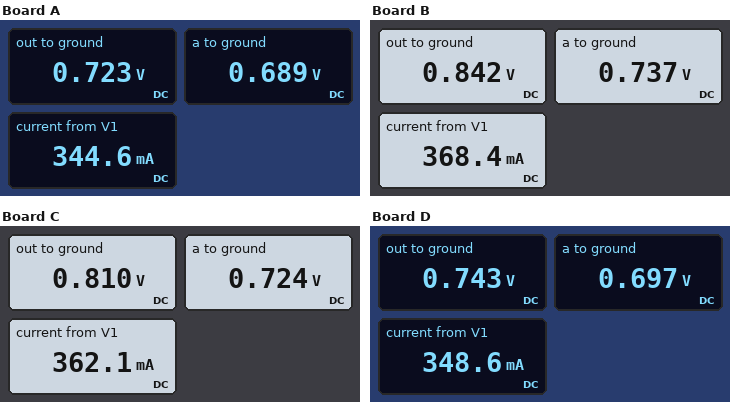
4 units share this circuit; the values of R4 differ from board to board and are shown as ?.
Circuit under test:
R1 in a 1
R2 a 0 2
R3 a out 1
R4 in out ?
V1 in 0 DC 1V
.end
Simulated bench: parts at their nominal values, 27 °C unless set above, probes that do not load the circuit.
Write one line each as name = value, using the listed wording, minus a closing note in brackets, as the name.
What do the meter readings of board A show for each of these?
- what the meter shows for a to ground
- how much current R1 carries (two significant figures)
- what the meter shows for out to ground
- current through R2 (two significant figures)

what the meter shows for a to ground = 0.689 V
how much current R1 carries = 310 mA
what the meter shows for out to ground = 0.723 V
current through R2 = 340 mA
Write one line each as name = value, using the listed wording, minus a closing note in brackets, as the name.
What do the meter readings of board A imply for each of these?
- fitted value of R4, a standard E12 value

fitted value of R4, a standard E12 value = 8.2 Ω
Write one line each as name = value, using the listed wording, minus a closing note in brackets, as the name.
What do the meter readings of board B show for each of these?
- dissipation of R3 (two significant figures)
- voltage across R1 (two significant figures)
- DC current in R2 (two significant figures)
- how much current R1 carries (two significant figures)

dissipation of R3 = 11 mW
voltage across R1 = 260 mV
DC current in R2 = 370 mA
how much current R1 carries = 260 mA
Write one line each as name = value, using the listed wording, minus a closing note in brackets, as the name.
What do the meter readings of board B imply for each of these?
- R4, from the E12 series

R4, from the E12 series = 1.5 Ω
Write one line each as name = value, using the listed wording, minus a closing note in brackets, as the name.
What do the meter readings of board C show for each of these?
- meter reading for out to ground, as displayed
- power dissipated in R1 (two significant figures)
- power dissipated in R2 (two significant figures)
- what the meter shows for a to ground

meter reading for out to ground, as displayed = 0.810 V
power dissipated in R1 = 76 mW
power dissipated in R2 = 260 mW
what the meter shows for a to ground = 0.724 V
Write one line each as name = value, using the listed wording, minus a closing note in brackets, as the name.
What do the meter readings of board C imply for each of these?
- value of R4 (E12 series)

value of R4 = 2.2 Ω
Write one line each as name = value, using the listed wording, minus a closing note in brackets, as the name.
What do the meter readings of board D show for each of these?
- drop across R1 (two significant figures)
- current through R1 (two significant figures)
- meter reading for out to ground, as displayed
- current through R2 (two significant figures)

drop across R1 = 300 mV
current through R1 = 300 mA
meter reading for out to ground, as displayed = 0.743 V
current through R2 = 350 mA
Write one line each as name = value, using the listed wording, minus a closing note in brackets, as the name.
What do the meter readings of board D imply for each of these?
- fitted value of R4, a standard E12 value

fitted value of R4, a standard E12 value = 5.6 Ω
